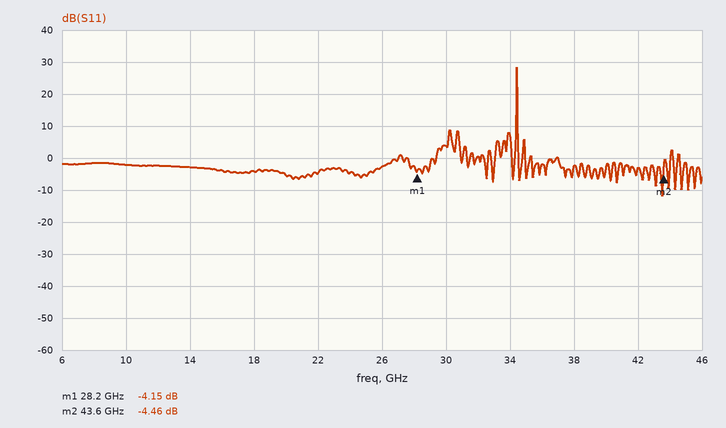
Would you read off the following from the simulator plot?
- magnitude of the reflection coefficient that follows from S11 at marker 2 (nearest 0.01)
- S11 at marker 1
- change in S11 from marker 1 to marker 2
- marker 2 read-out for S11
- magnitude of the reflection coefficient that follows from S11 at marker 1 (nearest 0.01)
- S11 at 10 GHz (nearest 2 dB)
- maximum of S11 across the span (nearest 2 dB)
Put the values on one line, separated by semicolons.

0.60; -4.15 dB; -0.31 dB; -4.46 dB; 0.62; -2 dB; 28 dB
